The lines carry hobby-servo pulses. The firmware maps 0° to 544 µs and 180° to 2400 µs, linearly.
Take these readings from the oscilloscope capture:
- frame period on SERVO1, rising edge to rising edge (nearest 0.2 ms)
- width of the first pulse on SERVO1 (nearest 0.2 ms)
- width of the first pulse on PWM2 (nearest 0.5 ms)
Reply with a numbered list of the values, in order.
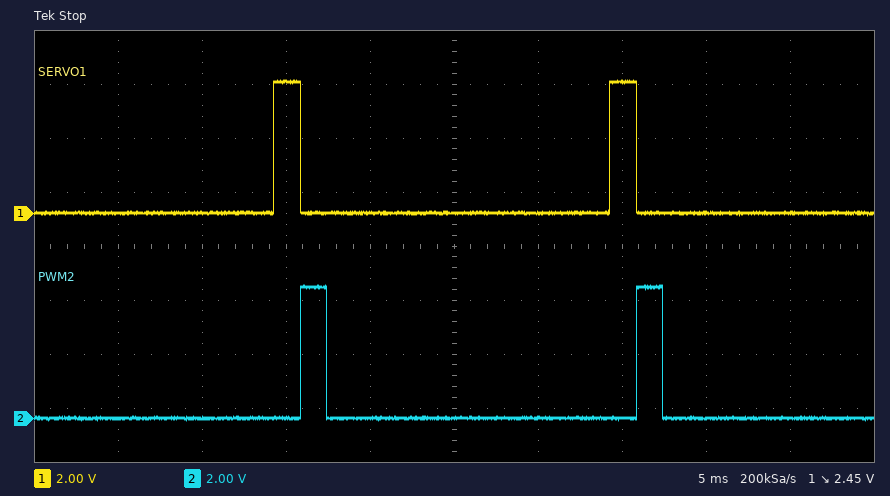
1. 20.0 ms
2. 1.6 ms
3. 1.5 ms
